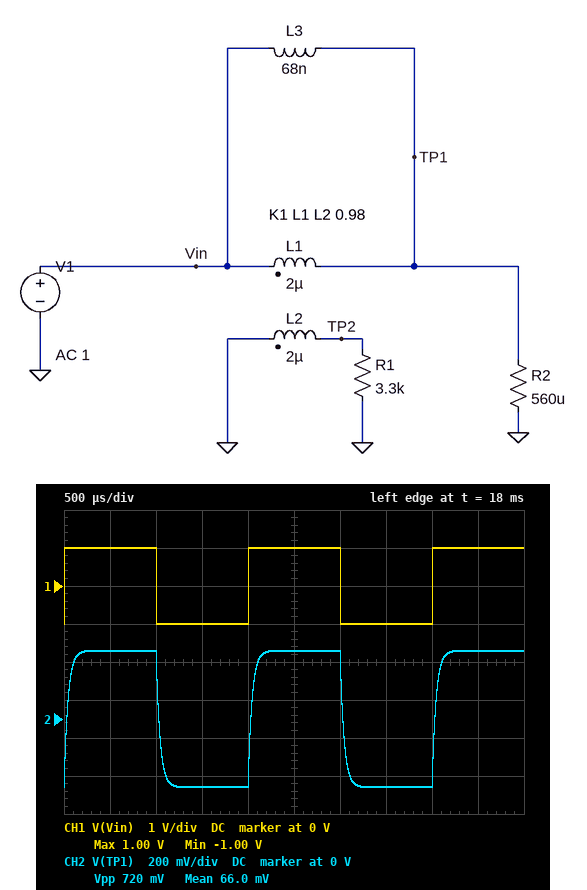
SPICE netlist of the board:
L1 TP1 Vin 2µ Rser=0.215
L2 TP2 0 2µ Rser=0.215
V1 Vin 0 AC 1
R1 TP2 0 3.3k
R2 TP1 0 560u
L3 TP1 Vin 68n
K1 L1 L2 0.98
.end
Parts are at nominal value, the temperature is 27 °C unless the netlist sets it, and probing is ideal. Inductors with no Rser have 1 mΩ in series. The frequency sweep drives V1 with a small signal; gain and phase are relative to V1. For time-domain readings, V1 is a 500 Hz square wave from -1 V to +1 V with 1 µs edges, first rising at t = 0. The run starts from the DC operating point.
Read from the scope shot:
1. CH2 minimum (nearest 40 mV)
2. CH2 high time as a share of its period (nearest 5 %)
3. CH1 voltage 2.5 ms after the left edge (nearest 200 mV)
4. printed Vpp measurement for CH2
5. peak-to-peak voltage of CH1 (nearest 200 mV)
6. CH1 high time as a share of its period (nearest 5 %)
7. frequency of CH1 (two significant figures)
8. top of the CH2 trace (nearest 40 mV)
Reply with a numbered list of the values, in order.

1. -360 mV
2. 50 %
3. 1.0 V
4. 720 mV
5. 2.0 V
6. 50 %
7. 500 Hz
8. 360 mV
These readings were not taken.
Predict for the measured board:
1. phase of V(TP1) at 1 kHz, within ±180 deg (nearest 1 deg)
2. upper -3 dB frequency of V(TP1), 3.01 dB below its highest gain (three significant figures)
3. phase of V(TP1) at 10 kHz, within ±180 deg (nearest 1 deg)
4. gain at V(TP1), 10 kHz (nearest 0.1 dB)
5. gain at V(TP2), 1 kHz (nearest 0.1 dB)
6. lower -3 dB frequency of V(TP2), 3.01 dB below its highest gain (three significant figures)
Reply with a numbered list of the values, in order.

1. -15 deg
2. 3.66 kHz
3. -69 deg
4. -18.1 dB
5. -28.3 dB
6. 17.6 kHz
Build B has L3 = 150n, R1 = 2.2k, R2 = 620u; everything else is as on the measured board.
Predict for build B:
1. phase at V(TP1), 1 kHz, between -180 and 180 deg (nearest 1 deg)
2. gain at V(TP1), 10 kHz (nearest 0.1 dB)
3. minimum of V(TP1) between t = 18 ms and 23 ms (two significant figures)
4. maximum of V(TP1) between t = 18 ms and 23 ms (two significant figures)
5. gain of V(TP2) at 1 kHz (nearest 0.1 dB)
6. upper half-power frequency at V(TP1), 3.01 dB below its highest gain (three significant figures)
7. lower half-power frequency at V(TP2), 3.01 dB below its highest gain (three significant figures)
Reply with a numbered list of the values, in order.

1. -30 deg
2. -23.6 dB
3. -380 mV
4. 380 mV
5. -27.6 dB
6. 1.72 kHz
7. 17.3 kHz
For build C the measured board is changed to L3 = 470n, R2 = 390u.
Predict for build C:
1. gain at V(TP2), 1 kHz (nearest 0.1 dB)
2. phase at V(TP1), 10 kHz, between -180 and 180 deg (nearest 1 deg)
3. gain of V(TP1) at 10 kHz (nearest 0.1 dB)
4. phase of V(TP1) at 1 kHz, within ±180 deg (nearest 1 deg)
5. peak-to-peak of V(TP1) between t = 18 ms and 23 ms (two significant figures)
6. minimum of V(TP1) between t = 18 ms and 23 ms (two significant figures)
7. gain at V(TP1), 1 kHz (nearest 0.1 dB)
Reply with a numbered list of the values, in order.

1. -25.3 dB
2. -82 deg
3. -37.0 dB
4. -64 deg
5. 510 mV
6. -250 mV
7. -18.4 dB
